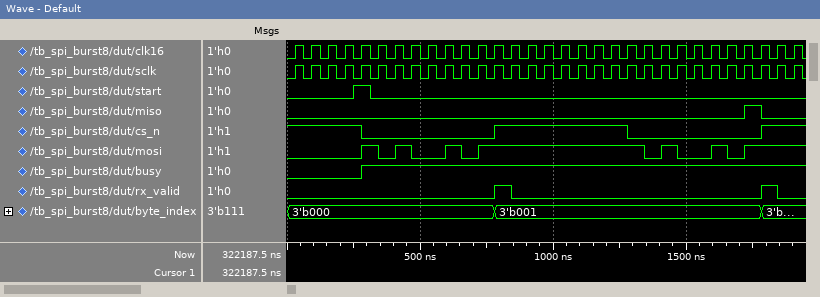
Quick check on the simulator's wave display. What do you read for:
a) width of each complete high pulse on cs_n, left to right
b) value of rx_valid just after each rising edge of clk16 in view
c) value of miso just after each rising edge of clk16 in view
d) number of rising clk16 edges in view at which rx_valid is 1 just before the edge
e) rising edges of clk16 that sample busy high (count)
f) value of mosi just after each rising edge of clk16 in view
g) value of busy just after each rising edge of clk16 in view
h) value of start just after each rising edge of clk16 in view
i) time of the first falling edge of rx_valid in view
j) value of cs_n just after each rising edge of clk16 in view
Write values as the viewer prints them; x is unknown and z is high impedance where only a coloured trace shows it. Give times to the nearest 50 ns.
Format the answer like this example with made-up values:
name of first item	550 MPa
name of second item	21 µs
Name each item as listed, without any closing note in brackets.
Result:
width of each complete high pulse on cs_n, left to right	500 ns
value of rx_valid just after each rising edge of clk16 in view	0 0 0 0 0 0 0 0 0 0 0 0 1 0 0 0 0 0 0 0 0 0 0 0 0 0 0 0 1 0 0
value of miso just after each rising edge of clk16 in view	0 0 0 0 0 0 0 0 0 0 0 0 0 0 0 0 0 0 0 0 0 0 0 0 0 0 0 1 0 0 0
number of rising clk16 edges in view at which rx_valid is 1 just before the edge	2
rising edges of clk16 that sample busy high	26
value of mosi just after each rising edge of clk16 in view	0 0 0 0 1 0 1 0 0 1 0 1 1 1 1 1 1 1 1 1 1 0 1 0 0 1 0 1 1 1 1
value of busy just after each rising edge of clk16 in view	0 0 0 0 1 1 1 1 1 1 1 1 1 1 1 1 1 1 1 1 1 1 1 1 1 1 1 1 1 1 1
value of start just after each rising edge of clk16 in view	0 0 0 0 1 0 0 0 0 0 0 0 0 0 0 0 0 0 0 0 0 0 0 0 0 0 0 0 0 0 0
time of the first falling edge of rx_valid in view	850 ns
value of cs_n just after each rising edge of clk16 in view	1 1 1 1 0 0 0 0 0 0 0 0 1 1 1 1 1 1 1 1 0 0 0 0 0 0 0 0 1 1 1
